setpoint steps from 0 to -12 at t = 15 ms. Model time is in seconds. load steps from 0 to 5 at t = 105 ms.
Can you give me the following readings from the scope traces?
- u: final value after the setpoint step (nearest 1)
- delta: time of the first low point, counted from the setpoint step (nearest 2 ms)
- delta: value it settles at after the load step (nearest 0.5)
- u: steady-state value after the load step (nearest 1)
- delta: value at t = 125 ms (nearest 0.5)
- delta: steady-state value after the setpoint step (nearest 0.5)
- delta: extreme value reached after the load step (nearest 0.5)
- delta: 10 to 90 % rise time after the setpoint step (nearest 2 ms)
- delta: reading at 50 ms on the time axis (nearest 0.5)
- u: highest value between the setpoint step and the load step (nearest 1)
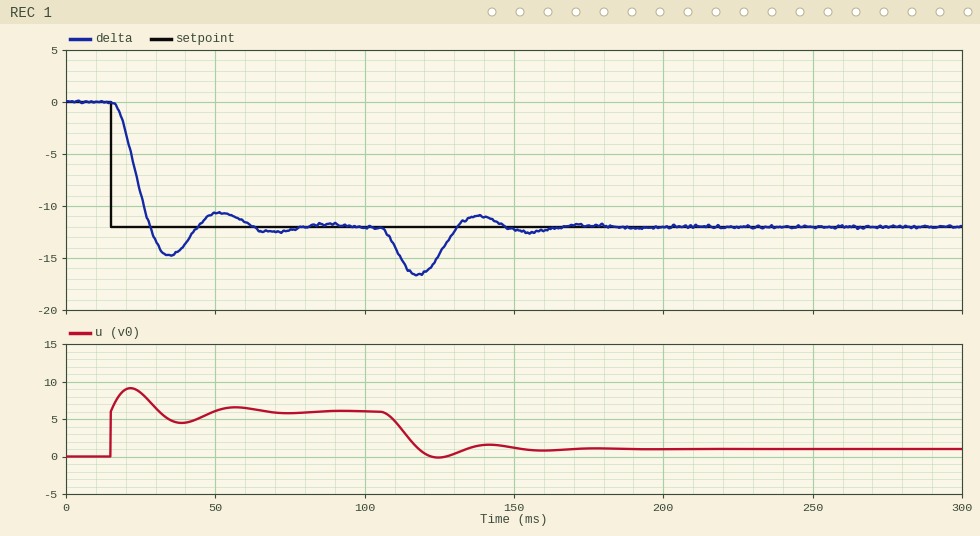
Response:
6
20 ms
-12.0
1
-14.5
-12.0
-16.5
8 ms
-10.5
9
